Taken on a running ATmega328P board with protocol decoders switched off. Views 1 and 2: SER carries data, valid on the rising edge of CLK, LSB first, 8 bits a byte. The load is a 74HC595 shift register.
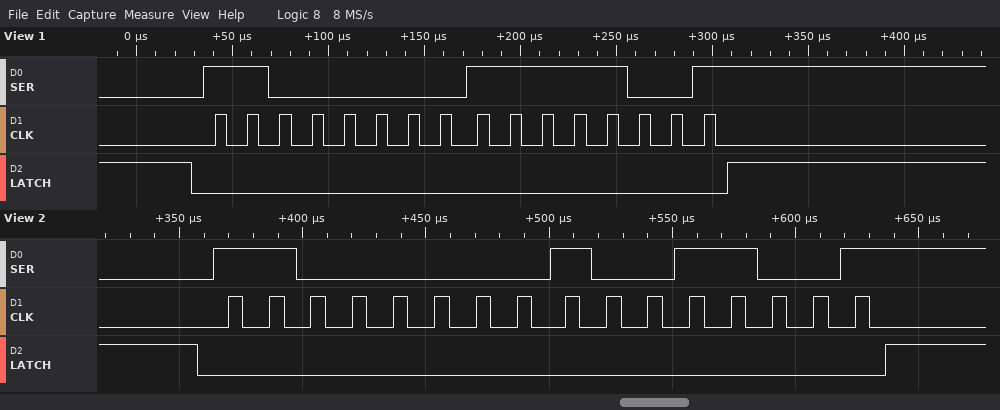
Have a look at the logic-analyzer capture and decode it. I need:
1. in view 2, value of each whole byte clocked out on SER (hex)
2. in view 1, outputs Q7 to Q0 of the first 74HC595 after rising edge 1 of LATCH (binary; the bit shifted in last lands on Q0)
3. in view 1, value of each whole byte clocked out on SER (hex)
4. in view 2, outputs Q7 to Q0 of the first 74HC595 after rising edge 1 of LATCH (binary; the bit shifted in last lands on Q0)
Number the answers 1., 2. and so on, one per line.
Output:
1. 03 99
2. 11111001
3. 03 9F
4. 10011001
